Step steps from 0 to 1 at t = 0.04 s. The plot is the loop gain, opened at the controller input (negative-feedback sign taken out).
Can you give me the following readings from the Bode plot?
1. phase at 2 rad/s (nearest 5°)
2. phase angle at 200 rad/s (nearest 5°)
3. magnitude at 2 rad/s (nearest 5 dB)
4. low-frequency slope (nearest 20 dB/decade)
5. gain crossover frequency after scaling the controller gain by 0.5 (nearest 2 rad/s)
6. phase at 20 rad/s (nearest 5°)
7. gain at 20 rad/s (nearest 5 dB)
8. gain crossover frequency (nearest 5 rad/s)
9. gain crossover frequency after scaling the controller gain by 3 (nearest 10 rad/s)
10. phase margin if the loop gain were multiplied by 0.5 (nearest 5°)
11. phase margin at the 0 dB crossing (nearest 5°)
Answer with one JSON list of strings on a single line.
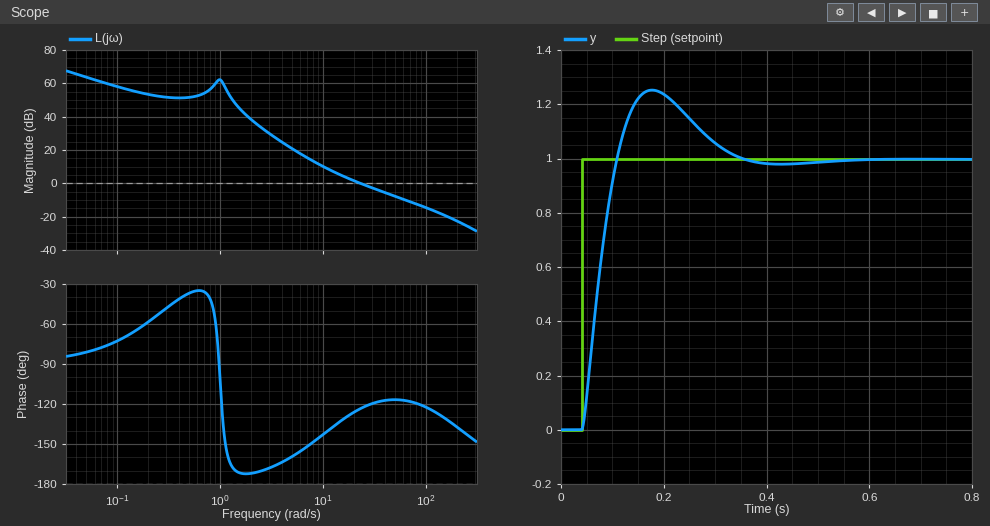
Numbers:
["-170°", "-135°", "40 dB", "-20 dB/decade", "14 rad/s", "-125°", "0 dB", "25 rad/s", "60 rad/s", "45°", "55°"]
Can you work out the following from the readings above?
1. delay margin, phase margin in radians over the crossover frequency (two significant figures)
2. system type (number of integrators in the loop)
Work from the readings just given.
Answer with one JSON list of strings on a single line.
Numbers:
["0.038 s", "1"]
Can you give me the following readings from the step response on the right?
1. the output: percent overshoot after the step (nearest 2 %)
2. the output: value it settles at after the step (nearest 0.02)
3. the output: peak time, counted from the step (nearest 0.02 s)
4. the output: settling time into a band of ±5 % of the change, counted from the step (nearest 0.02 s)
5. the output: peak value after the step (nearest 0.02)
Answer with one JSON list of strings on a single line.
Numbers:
["26 %", "1.00", "0.14 s", "0.26 s", "1.26"]
